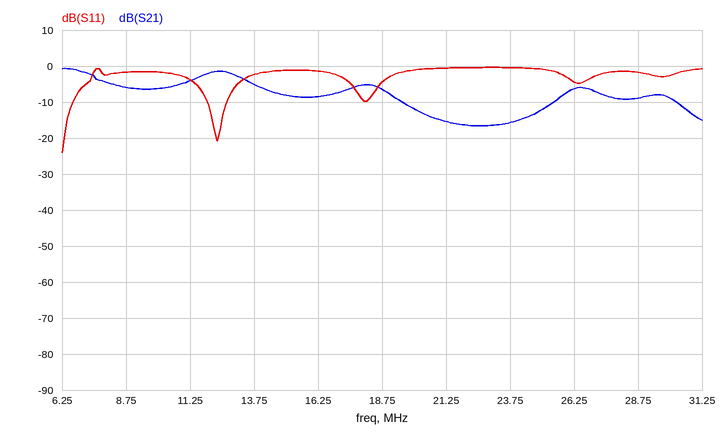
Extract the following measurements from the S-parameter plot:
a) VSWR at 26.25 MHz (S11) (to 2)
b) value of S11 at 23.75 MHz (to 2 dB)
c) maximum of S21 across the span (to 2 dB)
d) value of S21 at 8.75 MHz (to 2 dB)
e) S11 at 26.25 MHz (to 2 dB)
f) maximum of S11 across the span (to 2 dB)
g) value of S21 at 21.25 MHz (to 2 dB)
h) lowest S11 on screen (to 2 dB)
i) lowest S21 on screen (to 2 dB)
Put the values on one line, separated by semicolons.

4; 0 dB; 0 dB; -6 dB; -4 dB; 0 dB; -16 dB; -24 dB; -16 dB
